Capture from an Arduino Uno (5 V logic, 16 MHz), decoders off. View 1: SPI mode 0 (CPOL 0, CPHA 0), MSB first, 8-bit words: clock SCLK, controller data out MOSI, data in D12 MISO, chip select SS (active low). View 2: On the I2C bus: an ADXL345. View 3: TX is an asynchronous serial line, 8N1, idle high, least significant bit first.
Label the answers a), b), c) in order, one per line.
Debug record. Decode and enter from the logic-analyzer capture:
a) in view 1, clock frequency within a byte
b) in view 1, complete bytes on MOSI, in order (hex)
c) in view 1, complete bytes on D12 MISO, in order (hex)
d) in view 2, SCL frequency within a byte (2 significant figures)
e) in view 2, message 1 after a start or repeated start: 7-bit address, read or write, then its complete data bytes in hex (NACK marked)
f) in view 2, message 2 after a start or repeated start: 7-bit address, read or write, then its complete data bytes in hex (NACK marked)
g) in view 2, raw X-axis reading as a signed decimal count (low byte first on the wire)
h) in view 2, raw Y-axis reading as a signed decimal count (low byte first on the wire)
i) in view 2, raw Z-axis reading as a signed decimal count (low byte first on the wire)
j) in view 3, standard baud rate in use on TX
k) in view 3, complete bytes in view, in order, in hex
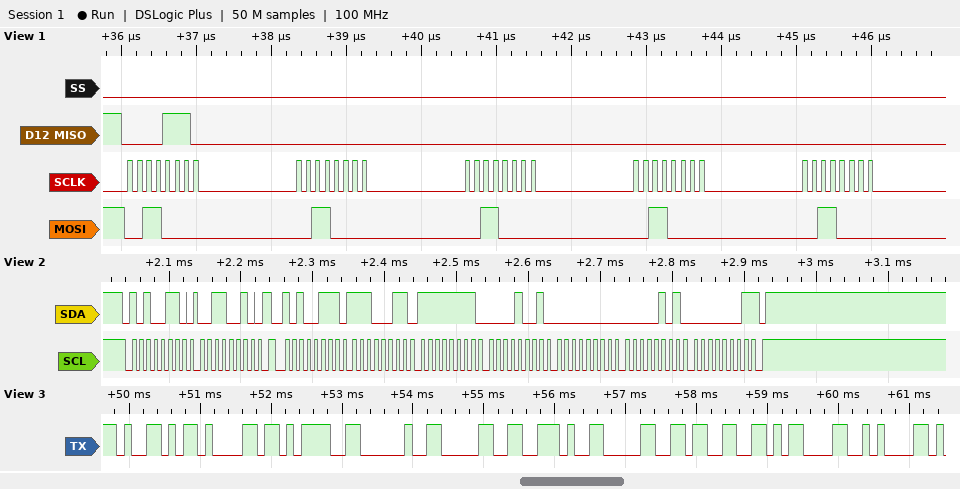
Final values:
a) 8 MHz
b) 30 30 30 30 30
c) 0E 00 00 00 00
d) 100 kHz
e) 0x53 write: 32
f) 0x53 read: E3 FF 09 00 05 01 NACK
g) -29
h) 9
i) 261
j) 9600 baud
k) 59 61 3D 20 30 2E 30 33 0D 0A
